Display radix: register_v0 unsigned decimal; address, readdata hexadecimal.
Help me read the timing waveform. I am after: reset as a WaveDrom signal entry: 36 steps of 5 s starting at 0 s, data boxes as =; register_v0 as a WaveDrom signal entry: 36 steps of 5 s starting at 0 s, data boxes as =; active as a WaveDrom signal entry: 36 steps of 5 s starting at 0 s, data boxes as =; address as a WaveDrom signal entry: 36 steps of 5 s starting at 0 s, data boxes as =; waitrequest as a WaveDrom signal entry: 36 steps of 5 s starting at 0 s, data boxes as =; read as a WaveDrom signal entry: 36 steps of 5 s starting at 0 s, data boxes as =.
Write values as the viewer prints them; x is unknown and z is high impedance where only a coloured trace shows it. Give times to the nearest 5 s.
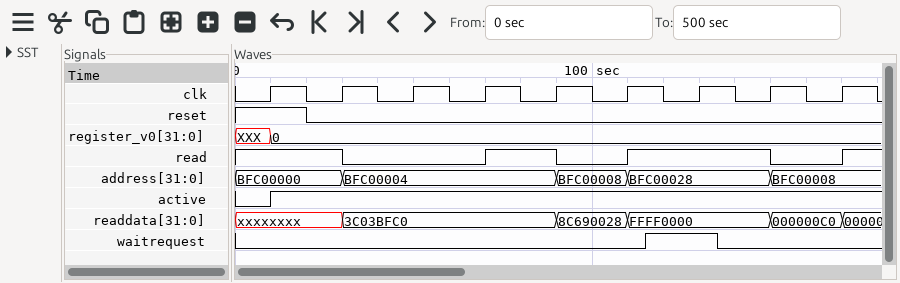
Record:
{name: 'reset', wave: '1...0...............................'}
{name: 'register_v0', wave: 'x.=.................................', data: '0'}
{name: 'active', wave: '0.1.................................'}
{name: 'address', wave: '=.....=...........=...=.......=.....', data: 'BFC00000 BFC00004 BFC00008 BFC00028 BFC00008'}
{name: 'waitrequest', wave: '0......................1...0........'}
{name: 'read', wave: '1.....0.......1...0...1.......0...1.'}
